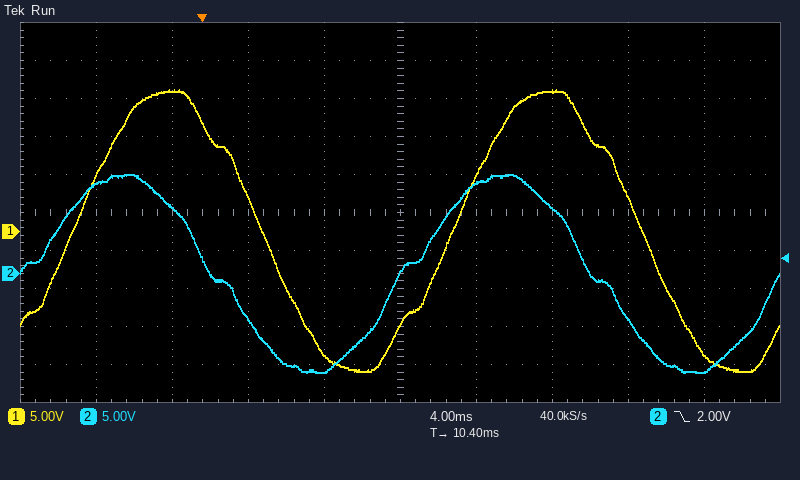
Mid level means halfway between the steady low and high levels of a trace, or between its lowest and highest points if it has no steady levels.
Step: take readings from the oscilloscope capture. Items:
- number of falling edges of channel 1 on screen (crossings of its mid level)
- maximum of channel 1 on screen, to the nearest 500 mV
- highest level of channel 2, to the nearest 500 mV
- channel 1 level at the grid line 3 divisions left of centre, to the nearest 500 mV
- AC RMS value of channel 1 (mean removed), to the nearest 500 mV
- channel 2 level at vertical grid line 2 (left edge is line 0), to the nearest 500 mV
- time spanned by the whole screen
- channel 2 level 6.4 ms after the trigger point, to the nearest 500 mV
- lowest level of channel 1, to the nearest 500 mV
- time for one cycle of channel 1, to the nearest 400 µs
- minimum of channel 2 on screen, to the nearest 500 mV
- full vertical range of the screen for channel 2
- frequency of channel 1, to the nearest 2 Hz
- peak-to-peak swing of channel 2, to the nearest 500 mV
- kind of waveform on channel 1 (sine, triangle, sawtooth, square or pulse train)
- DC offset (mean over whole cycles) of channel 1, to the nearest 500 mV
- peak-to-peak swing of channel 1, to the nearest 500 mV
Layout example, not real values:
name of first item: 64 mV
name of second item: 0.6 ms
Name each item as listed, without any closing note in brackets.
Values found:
number of falling edges of channel 1 on screen: 2
maximum of channel 1 on screen, to the nearest 500 mV: 18.5 V
highest level of channel 2, to the nearest 500 mV: 13.0 V
channel 1 level at the grid line 3 divisions left of centre, to the nearest 500 mV: 18.5 V
AC RMS value of channel 1 (mean removed), to the nearest 500 mV: 13.0 V
channel 2 level at vertical grid line 2 (left edge is line 0), to the nearest 500 mV: 8.5 V
time spanned by the whole screen: 40 ms
channel 2 level 6.4 ms after the trigger point, to the nearest 500 mV: -13.0 V
lowest level of channel 1, to the nearest 500 mV: -18.5 V
time for one cycle of channel 1, to the nearest 400 µs: 20.0 ms
minimum of channel 2 on screen, to the nearest 500 mV: -13.0 V
full vertical range of the screen for channel 2: 50 V
frequency of channel 1, to the nearest 2 Hz: 50 Hz
peak-to-peak swing of channel 2, to the nearest 500 mV: 26.0 V
kind of waveform on channel 1: sine
DC offset (mean over whole cycles) of channel 1, to the nearest 500 mV: 0.0 V
peak-to-peak swing of channel 1, to the nearest 500 mV: 37.0 V
